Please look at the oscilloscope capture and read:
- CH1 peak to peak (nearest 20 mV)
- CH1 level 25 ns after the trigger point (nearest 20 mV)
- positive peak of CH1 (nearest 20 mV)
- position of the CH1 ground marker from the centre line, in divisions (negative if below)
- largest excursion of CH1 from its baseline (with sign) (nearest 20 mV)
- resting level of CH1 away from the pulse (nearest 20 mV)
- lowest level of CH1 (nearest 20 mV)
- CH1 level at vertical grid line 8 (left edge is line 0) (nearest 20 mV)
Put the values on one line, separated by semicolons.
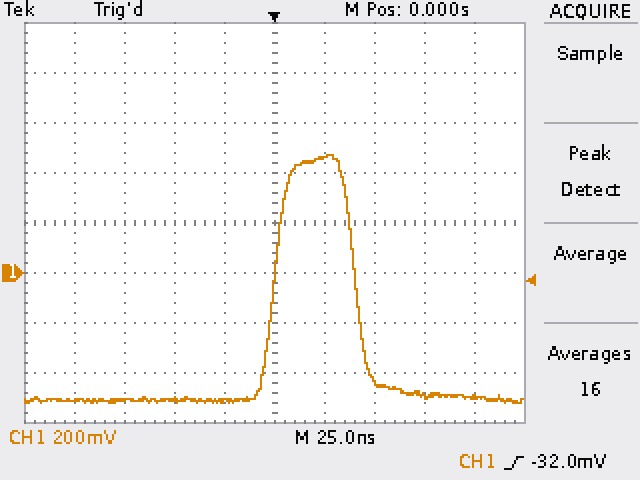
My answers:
1.00 V; 460 mV; 480 mV; -1.0 div; +980 mV; -500 mV; -520 mV; -500 mV
